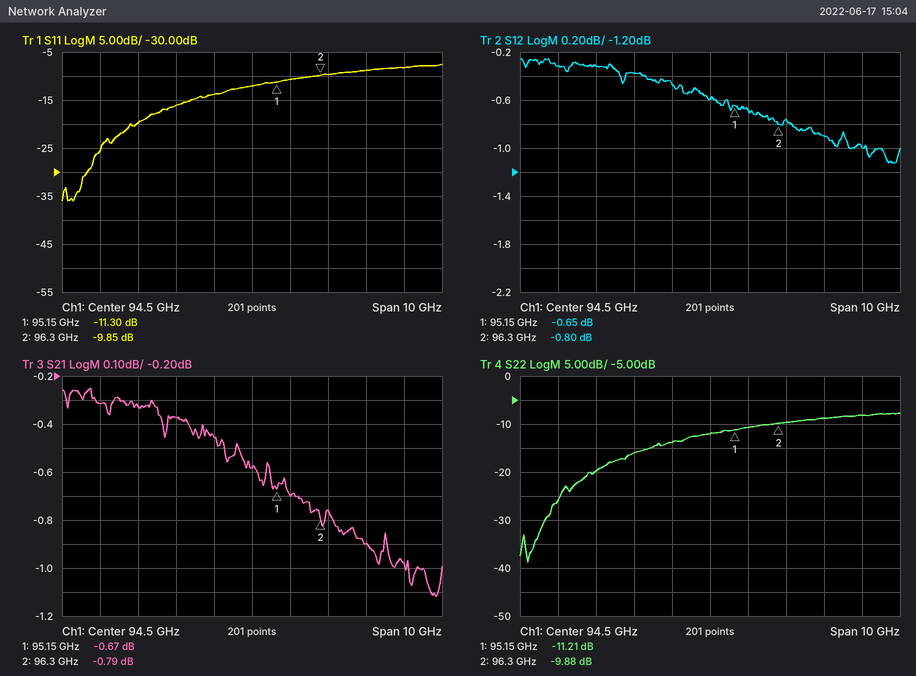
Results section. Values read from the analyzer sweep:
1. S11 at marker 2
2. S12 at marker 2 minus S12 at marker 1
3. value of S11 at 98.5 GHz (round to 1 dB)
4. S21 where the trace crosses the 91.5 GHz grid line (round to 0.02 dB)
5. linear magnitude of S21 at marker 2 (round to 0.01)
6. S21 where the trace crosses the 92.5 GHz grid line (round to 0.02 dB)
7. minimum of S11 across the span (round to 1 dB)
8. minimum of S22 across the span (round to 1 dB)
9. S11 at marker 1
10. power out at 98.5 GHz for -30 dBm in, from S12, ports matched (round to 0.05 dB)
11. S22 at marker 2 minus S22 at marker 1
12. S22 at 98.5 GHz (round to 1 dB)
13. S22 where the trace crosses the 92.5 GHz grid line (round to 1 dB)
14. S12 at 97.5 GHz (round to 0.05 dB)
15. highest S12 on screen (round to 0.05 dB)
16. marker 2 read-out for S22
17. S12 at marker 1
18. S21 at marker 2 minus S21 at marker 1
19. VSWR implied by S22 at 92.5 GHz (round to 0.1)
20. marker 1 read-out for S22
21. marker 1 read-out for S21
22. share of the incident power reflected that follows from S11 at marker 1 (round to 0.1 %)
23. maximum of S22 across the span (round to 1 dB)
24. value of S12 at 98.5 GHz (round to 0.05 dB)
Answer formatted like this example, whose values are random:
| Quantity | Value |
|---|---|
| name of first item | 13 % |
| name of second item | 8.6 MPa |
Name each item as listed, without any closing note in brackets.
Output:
| Quantity | Value |
|---|---|
| S11 at marker 2 | -9.85 dB |
| S12 at marker 2 minus S12 at marker 1 | -0.15 dB |
| value of S11 at 98.5 GHz | -8 dB |
| S21 where the trace crosses the 91.5 GHz grid line | -0.32 dB |
| linear magnitude of S21 at marker 2 | 0.91 |
| S21 where the trace crosses the 92.5 GHz grid line | -0.38 dB |
| minimum of S11 across the span | -36 dB |
| minimum of S22 across the span | -39 dB |
| S11 at marker 1 | -11.30 dB |
| power out at 98.5 GHz for -30 dBm in, from S12, ports matched | -31.00 dBm |
| S22 at marker 2 minus S22 at marker 1 | 1.33 dB |
| S22 at 98.5 GHz | -8 dB |
| S22 where the trace crosses the 92.5 GHz grid line | -16 dB |
| S12 at 97.5 GHz | -0.90 dB |
| highest S12 on screen | -0.25 dB |
| marker 2 read-out for S22 | -9.88 dB |
| S12 at marker 1 | -0.65 dB |
| S21 at marker 2 minus S21 at marker 1 | -0.12 dB |
| VSWR implied by S22 at 92.5 GHz | 1.4 |
| marker 1 read-out for S22 | -11.21 dB |
| marker 1 read-out for S21 | -0.67 dB |
| share of the incident power reflected that follows from S11 at marker 1 | 7.4 % |
| maximum of S22 across the span | -8 dB |
| value of S12 at 98.5 GHz | -1.00 dB |
